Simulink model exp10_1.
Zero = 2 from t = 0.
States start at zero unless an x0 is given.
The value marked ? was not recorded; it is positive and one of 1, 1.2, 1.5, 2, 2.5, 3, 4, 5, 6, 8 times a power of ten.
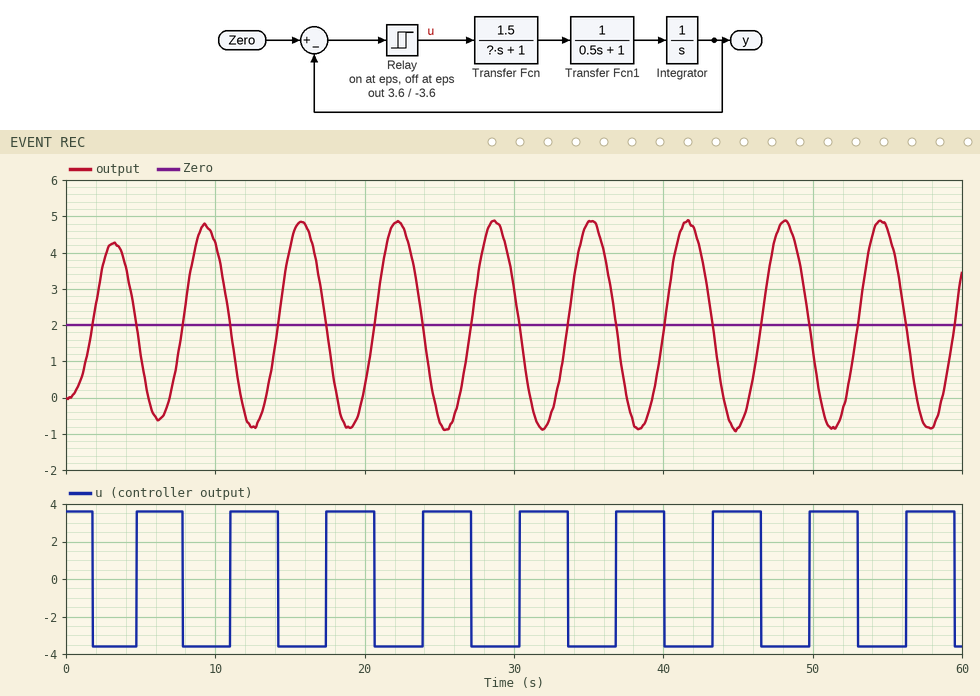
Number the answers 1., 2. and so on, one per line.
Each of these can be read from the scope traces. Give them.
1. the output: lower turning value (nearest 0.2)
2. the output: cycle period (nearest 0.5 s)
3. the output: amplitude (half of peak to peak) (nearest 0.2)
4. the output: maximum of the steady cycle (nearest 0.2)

1. -0.8
2. 6.5 s
3. 2.8
4. 4.8
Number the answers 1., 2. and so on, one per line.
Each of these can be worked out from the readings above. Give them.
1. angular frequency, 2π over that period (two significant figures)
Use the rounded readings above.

1. 0.97 rad/s
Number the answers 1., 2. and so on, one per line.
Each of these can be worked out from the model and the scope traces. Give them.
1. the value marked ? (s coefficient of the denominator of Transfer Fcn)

1. 2
